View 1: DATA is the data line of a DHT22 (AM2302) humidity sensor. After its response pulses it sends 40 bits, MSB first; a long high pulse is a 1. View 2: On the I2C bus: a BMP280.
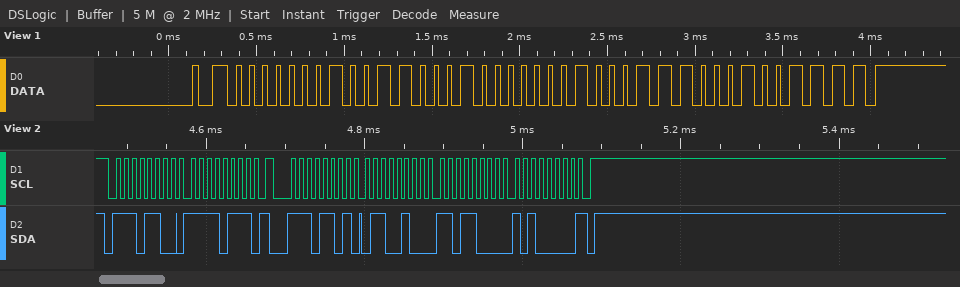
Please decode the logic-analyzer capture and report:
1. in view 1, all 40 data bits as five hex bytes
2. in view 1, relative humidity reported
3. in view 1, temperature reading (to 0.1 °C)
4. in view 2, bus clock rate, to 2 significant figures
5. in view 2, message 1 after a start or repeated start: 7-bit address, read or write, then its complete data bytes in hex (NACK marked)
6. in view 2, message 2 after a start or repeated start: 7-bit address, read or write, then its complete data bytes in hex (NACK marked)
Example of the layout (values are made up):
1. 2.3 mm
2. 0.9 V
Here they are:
1. 01 31 01 1C 4F
2. 30.5 %
3. 28.4 °C
4. 100 kHz
5. 0x76 write: F7
6. 0x76 read: 64 D8 A0 NACK
